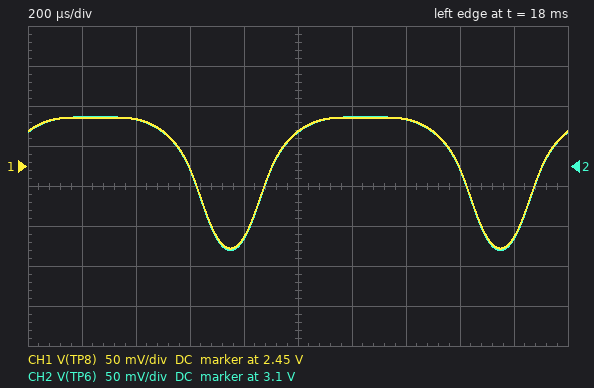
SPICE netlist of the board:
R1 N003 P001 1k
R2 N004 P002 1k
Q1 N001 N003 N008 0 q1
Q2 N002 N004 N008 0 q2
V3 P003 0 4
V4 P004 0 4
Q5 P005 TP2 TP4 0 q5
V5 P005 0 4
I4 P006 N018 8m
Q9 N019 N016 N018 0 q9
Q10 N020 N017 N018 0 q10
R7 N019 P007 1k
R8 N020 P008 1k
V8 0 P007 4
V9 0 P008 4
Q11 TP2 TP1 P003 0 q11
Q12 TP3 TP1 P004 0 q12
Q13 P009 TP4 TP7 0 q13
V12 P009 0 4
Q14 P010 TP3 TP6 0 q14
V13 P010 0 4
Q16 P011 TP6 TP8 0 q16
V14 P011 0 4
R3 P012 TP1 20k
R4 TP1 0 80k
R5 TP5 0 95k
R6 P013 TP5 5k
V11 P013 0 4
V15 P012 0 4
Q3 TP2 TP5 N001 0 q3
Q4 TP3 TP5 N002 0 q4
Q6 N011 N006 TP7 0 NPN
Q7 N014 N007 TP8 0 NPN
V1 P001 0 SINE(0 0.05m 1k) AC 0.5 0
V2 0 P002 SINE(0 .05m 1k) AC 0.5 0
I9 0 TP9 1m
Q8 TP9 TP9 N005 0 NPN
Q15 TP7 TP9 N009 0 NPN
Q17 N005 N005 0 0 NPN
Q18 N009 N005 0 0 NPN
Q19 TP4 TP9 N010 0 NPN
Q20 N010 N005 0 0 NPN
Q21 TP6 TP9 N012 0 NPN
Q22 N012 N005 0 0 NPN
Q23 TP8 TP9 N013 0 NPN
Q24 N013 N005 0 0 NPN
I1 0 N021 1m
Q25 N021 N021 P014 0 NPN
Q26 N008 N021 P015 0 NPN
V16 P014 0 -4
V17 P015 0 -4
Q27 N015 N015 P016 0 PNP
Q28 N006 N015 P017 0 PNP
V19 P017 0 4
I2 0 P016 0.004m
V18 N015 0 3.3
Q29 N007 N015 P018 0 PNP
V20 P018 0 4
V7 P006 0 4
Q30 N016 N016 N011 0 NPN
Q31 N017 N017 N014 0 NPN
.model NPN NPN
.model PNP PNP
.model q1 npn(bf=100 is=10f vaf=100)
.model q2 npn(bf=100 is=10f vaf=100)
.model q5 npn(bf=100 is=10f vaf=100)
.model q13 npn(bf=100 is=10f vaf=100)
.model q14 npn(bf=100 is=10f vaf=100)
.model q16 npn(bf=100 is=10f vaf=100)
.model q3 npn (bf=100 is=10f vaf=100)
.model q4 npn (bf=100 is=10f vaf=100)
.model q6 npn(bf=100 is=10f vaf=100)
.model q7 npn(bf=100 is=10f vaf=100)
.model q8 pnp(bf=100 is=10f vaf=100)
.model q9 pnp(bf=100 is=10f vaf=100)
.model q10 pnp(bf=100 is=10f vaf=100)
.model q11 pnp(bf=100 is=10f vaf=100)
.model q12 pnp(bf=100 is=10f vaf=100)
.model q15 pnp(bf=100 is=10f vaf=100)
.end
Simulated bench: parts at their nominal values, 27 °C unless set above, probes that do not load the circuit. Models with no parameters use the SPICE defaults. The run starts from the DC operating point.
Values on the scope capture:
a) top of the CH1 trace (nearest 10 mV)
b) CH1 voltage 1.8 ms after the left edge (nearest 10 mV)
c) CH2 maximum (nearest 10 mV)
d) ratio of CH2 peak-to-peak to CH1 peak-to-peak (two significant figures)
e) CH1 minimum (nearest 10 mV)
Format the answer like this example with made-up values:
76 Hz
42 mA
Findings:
2.51 V
2.36 V
3.16 V
1.0
2.35 V
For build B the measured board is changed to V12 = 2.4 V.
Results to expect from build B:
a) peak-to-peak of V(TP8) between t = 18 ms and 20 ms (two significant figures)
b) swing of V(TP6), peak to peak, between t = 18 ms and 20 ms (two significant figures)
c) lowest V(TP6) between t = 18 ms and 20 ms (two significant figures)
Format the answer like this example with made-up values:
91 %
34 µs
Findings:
2.7 mV
2.8 mV
3.2 V
